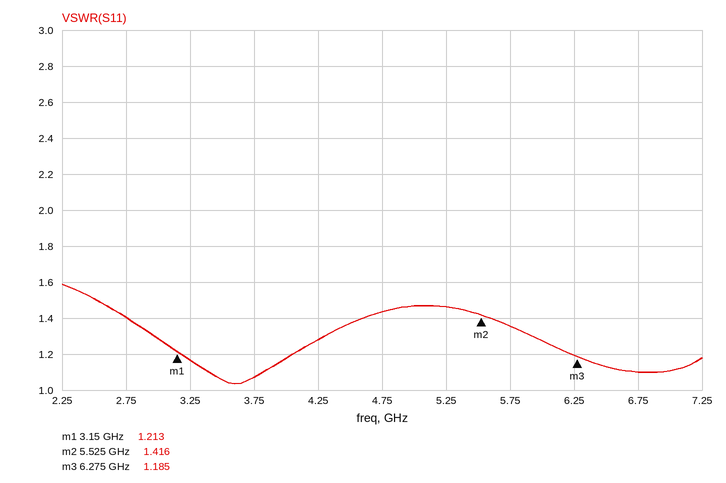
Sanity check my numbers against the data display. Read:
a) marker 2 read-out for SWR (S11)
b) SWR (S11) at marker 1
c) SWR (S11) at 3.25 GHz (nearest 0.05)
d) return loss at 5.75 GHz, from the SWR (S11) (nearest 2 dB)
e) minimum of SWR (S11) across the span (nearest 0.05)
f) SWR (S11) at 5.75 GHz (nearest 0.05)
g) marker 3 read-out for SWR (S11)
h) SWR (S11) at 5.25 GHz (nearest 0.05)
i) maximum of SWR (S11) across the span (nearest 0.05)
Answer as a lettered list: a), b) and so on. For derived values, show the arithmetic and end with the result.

a) 1.416
b) 1.213
c) 1.15
d) −20 log10((1.35 − 1)/(1.35 + 1)) ≈ 16 dB
e) 1.05
f) 1.35
g) 1.185
h) 1.45
i) 1.60
